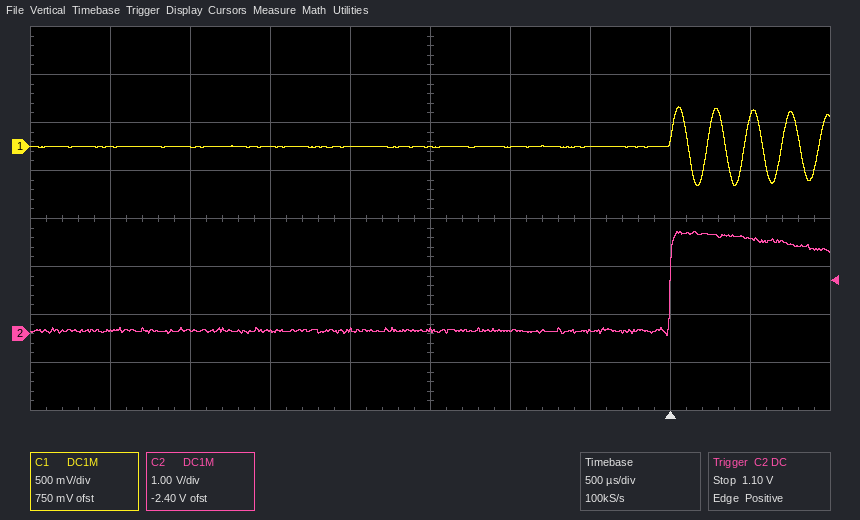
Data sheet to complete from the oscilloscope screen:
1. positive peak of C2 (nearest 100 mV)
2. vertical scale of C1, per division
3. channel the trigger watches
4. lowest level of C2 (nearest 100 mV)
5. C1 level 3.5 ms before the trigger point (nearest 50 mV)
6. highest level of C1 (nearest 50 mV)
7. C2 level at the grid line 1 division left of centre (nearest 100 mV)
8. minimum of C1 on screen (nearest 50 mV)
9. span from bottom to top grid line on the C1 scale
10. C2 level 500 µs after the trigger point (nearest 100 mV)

2.1 V
500 mV
C2
0.0 V
0 mV
400 mV
100 mV
-400 mV
4 V
2.0 V
